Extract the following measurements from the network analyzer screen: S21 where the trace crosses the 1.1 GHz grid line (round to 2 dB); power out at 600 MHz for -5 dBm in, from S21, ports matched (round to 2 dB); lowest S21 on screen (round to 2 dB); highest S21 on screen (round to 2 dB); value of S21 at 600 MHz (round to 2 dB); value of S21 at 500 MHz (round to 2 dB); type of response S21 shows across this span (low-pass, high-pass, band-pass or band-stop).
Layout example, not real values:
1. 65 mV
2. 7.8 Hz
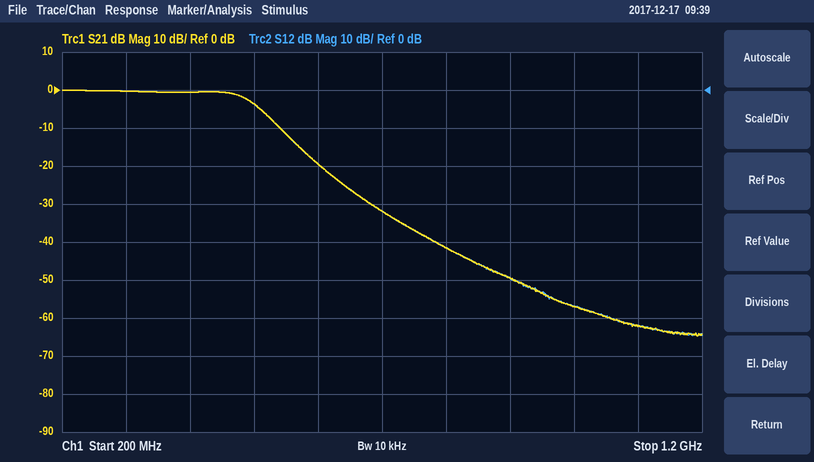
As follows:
1. -62 dB
2. -24 dBm
3. -64 dB
4. 0 dB
5. -20 dB
6. -4 dB
7. low-pass
